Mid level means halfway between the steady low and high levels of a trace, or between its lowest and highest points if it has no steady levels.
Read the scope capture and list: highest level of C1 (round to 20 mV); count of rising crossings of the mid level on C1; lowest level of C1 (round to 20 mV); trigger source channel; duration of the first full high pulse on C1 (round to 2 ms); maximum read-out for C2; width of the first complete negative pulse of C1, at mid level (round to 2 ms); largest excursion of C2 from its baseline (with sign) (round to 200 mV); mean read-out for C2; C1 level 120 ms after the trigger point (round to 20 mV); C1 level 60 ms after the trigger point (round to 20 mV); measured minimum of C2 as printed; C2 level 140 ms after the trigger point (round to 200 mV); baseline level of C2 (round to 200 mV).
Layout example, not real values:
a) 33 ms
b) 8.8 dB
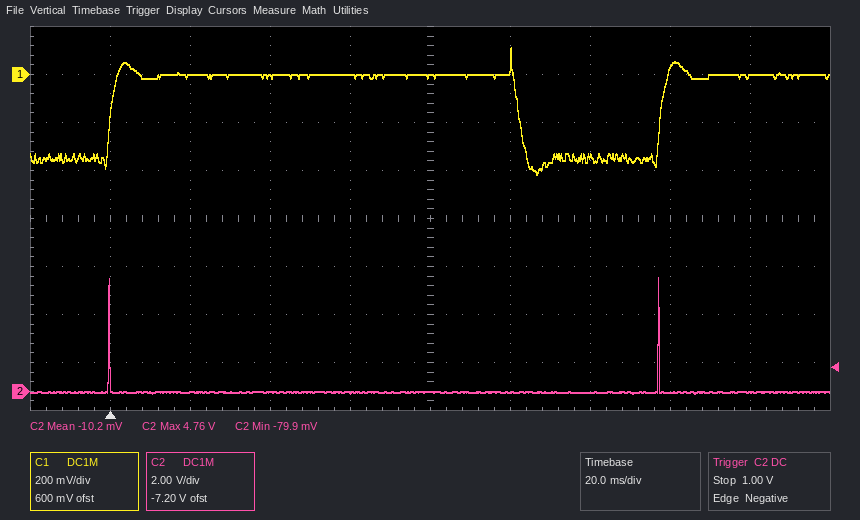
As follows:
a) 120 mV
b) 2
c) -420 mV
d) C2
e) 102 ms
f) 4.76 V
g) 36 ms
h) +4.8 V
i) -10.2 mV
j) -340 mV
k) 0 mV
l) -79.9 mV
m) 0.0 V
n) 0.0 V
